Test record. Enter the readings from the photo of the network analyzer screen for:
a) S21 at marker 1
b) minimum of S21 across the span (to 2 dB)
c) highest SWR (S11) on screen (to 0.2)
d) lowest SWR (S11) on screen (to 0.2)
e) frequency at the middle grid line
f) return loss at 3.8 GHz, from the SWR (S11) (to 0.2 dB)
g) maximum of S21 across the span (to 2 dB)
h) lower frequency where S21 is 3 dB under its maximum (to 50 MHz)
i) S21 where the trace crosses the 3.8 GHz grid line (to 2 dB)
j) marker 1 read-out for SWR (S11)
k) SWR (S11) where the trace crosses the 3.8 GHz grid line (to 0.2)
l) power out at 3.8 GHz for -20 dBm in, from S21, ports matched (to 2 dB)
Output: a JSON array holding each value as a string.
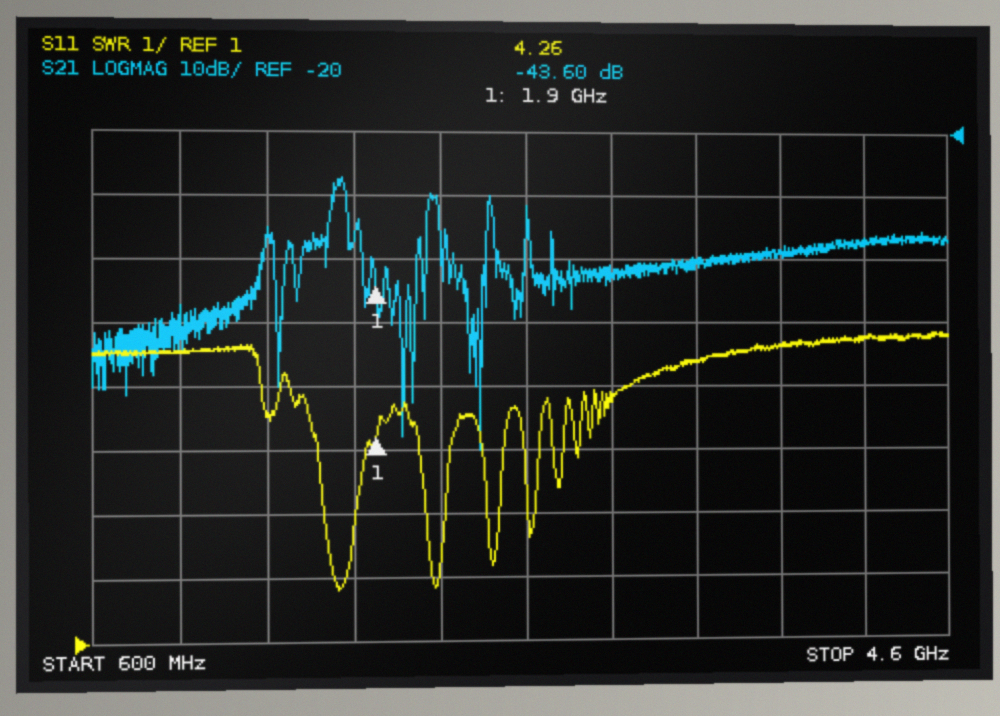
["-43.60 dB", "-70 dB", "5.8", "1.8", "2.6 GHz", "3.2 dB", "-28 dB", "1.70 GHz", "-38 dB", "4.26", "5.6", "-58 dBm"]
